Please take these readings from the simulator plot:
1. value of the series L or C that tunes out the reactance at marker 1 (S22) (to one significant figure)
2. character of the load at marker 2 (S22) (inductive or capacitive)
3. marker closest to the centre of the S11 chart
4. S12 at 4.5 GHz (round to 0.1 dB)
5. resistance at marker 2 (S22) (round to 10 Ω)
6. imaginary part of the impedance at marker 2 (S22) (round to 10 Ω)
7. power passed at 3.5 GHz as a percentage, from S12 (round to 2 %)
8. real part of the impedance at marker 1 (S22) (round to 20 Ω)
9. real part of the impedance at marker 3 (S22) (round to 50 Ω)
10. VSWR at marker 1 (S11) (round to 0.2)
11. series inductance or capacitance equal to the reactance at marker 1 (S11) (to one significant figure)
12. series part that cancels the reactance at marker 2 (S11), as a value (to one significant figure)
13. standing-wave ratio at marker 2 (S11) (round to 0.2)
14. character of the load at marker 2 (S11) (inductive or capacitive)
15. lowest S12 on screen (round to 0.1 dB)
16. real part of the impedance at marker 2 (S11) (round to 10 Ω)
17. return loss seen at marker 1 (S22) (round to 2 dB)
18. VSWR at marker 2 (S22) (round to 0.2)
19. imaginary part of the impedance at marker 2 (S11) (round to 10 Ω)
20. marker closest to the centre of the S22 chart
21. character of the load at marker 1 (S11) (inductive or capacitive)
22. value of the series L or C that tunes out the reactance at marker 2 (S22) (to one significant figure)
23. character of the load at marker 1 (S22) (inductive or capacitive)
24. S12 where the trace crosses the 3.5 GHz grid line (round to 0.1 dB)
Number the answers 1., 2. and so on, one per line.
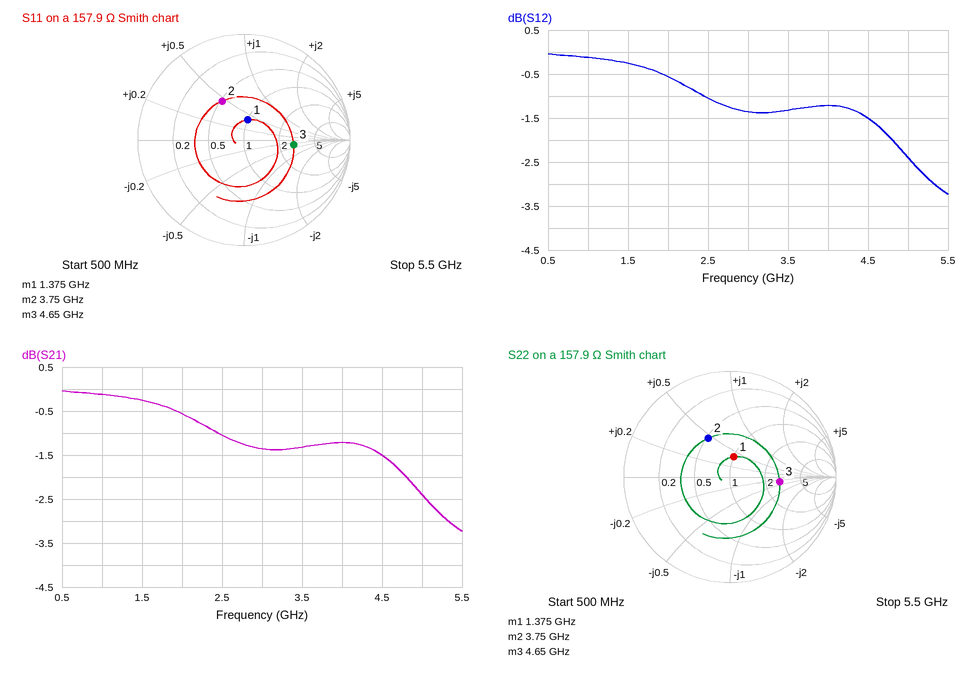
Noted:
1. 2 pF
2. inductive
3. marker 1
4. -1.5 dB
5. 80 Ω
6. +70 Ω
7. 74 %
8. 160 Ω
9. 450 Ω
10. 1.4
11. 7 nH
12. 600 fF
13. 2.4
14. inductive
15. -3.2 dB
16. 80 Ω
17. 14 dB
18. 2.4
19. +70 Ω
20. marker 1
21. inductive
22. 600 fF
23. inductive
24. -1.3 dB
